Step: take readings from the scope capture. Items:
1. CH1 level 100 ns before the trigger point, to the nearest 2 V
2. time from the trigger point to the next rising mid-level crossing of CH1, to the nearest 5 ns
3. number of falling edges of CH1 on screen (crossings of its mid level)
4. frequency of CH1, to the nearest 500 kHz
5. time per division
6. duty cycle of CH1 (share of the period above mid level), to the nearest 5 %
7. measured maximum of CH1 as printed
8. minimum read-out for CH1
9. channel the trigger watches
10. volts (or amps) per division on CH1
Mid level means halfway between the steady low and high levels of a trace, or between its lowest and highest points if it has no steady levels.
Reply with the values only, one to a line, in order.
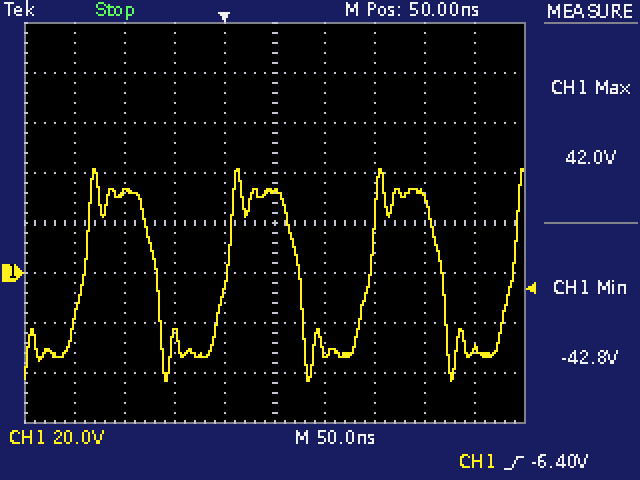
32 V
5 ns
3
7.0 MHz
50 ns
50 %
42.0 V
-42.8 V
CH1
20 V
